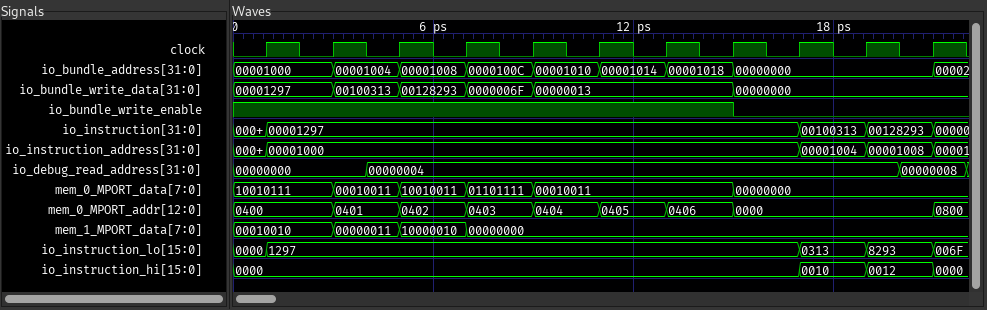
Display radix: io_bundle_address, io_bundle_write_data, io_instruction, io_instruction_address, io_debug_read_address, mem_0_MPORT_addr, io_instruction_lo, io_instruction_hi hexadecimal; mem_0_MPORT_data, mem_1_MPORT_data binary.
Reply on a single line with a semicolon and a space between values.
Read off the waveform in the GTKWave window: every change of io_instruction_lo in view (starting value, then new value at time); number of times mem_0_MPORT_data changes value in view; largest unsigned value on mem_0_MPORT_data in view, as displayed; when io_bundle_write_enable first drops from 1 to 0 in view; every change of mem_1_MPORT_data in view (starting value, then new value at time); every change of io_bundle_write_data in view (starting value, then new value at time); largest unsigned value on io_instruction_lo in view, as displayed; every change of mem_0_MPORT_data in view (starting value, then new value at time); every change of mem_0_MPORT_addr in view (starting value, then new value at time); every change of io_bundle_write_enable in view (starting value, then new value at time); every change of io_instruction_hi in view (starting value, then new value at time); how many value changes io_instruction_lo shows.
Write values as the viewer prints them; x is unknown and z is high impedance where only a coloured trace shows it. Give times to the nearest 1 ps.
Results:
0000, 1297 at 1 ps, 0313 at 17 ps, 8293 at 19 ps, 006F at 21 ps; 5; 10010111; 15 ps; 00010010, 00000011 at 3 ps, 10000010 at 5 ps, 00000000 at 7 ps; 00001297, 00100313 at 3 ps, 00128293 at 5 ps, 0000006F at 7 ps, 00000013 at 9 ps, 00000000 at 15 ps; 8293; 10010111, 00010011 at 3 ps, 10010011 at 5 ps, 01101111 at 7 ps, 00010011 at 9 ps, 00000000 at 15 ps; 0400, 0401 at 3 ps, 0402 at 5 ps, 0403 at 7 ps, 0404 at 9 ps, 0405 at 11 ps, 0406 at 13 ps, 0000 at 15 ps, 0800 at 21 ps; 1, 0 at 15 ps; 0000, 0010 at 17 ps, 0012 at 19 ps, 0000 at 21 ps; 4
